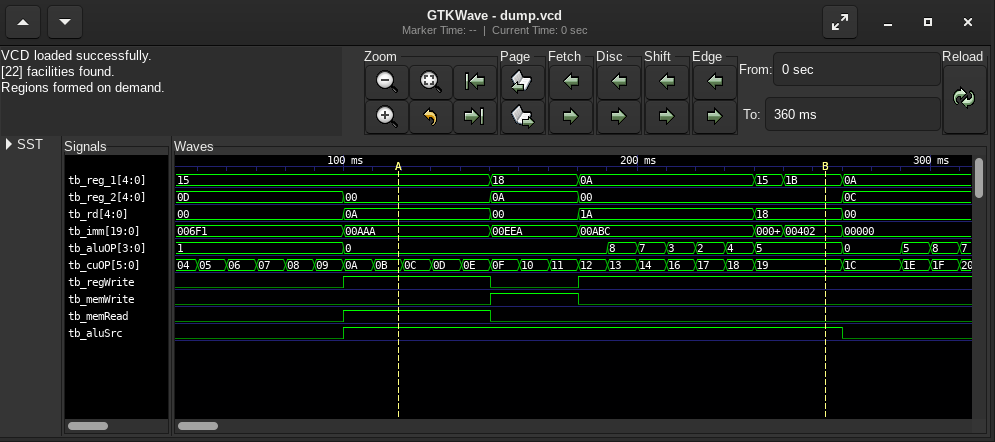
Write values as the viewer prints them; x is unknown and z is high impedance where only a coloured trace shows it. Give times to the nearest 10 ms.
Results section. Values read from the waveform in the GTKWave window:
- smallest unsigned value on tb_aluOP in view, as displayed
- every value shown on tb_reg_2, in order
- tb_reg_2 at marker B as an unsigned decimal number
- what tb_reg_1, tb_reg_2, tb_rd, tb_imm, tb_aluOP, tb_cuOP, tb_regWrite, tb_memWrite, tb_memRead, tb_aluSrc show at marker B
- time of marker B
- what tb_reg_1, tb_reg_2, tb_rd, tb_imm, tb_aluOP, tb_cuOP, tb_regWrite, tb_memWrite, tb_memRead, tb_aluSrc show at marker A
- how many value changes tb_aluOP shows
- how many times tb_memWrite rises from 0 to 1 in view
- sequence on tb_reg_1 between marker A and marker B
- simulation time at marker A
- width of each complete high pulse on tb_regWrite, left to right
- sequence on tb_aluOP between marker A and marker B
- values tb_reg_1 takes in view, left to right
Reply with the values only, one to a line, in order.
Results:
0
0D, 00, 0A, 00, 0C
0
tb_reg_1=1B, tb_reg_2=00, tb_rd=18, tb_imm=00402, tb_aluOP=5, tb_cuOP=19, tb_regWrite=1, tb_memWrite=0, tb_memRead=0, tb_aluSrc=1
260 ms
tb_reg_1=15, tb_reg_2=00, tb_rd=0A, tb_imm=00AAA, tb_aluOP=0, tb_cuOP=0B, tb_regWrite=1, tb_memWrite=0, tb_memRead=1, tb_aluSrc=1
11
1
15, 18, 0A, 15, 1B
120 ms
50 ms
0, 8, 7, 3, 2, 4, 5
15, 18, 0A, 15, 1B, 0A
